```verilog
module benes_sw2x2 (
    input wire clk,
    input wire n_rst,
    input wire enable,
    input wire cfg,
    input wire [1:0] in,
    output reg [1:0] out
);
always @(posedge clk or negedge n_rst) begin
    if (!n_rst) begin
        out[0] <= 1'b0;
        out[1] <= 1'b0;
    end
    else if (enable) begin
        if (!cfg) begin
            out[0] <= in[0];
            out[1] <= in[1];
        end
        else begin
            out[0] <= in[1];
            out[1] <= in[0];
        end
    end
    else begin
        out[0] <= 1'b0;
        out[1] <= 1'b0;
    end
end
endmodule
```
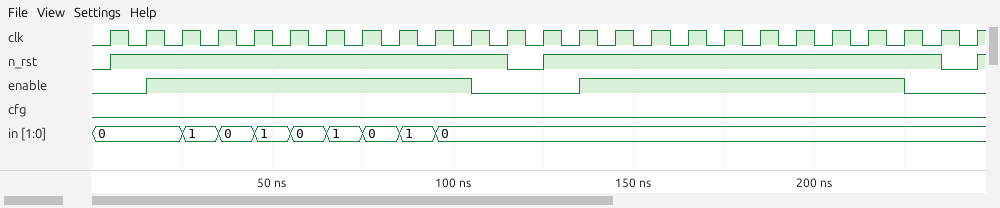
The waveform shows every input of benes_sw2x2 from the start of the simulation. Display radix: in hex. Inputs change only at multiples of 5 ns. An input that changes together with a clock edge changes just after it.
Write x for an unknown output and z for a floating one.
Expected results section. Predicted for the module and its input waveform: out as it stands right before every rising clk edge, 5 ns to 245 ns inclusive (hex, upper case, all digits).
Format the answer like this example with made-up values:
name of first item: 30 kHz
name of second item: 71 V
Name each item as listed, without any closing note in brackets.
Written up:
out as it stands right before every rising clk edge, 5 ns to 245 ns inclusive: 0, 0, 0, 0, 1, 0, 1, 0, 1, 0, 1, 0, 0, 0, 0, 0, 0, 0, 0, 0, 0, 0, 0, 0, 0
